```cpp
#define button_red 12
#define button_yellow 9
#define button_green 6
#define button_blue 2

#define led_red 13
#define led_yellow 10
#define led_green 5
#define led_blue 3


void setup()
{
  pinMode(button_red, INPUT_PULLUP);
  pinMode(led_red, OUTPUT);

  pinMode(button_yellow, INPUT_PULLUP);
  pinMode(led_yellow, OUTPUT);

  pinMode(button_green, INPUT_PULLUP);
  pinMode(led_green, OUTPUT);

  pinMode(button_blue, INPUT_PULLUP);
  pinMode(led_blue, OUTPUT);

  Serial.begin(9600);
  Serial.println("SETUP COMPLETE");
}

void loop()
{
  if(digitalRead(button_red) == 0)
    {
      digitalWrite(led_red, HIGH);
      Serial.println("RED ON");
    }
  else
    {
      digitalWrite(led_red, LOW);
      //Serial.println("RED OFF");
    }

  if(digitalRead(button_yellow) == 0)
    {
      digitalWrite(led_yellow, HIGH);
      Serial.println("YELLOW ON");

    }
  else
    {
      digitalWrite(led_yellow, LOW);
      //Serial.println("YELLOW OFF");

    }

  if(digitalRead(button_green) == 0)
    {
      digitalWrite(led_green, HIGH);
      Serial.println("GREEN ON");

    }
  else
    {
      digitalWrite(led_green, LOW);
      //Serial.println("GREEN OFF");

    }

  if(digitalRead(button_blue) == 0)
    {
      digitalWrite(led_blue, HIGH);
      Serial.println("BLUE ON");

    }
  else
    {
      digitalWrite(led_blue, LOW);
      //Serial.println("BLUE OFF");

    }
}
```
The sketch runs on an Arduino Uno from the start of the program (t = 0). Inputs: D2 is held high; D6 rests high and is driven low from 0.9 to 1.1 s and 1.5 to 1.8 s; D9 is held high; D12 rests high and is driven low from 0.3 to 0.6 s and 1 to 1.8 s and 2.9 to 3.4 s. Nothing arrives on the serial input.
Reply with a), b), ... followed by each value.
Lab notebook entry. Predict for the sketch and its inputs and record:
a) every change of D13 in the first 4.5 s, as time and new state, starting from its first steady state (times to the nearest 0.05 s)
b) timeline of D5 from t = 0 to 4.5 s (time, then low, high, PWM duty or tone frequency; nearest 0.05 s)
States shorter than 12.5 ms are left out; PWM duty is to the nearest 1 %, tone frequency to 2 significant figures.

a) 0 s low; 0.3 s high; 0.6 s low; 1 s high; 1.8 s low; 2.9 s high; 3.4 s low
b) 0 s low; 0.9 s high; 1.1 s low; 1.5 s high; 1.8 s low
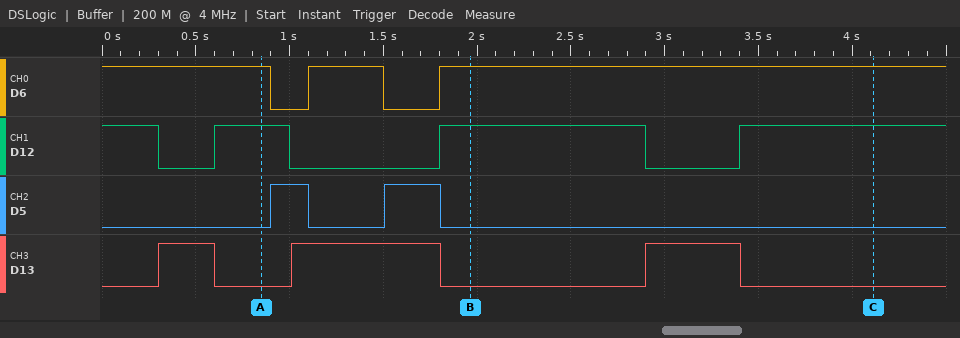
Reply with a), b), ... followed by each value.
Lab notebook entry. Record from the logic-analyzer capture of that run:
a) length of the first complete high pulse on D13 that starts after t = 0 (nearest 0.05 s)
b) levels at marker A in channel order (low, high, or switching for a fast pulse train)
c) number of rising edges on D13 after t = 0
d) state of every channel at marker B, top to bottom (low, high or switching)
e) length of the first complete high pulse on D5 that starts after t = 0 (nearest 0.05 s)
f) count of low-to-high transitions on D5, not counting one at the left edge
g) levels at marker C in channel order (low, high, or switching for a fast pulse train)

a) 0.30 s
b) D6 high, D12 high, D5 low, D13 low
c) 3
d) D6 high, D12 high, D5 low, D13 low
e) 0.20 s
f) 2
g) D6 high, D12 high, D5 low, D13 low
